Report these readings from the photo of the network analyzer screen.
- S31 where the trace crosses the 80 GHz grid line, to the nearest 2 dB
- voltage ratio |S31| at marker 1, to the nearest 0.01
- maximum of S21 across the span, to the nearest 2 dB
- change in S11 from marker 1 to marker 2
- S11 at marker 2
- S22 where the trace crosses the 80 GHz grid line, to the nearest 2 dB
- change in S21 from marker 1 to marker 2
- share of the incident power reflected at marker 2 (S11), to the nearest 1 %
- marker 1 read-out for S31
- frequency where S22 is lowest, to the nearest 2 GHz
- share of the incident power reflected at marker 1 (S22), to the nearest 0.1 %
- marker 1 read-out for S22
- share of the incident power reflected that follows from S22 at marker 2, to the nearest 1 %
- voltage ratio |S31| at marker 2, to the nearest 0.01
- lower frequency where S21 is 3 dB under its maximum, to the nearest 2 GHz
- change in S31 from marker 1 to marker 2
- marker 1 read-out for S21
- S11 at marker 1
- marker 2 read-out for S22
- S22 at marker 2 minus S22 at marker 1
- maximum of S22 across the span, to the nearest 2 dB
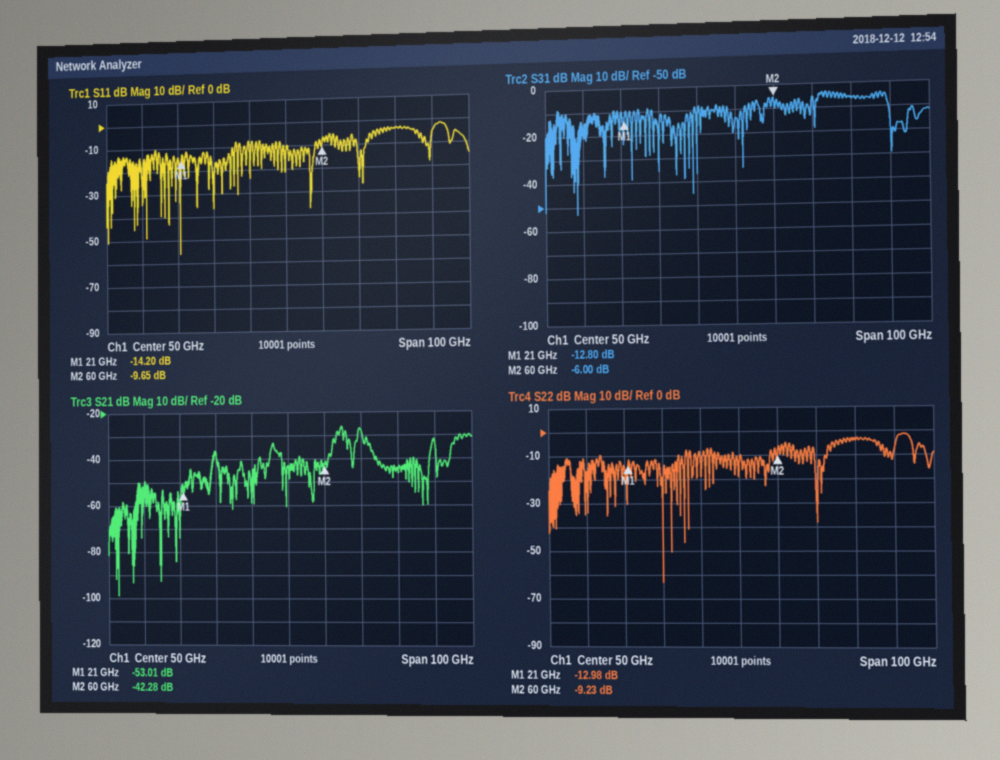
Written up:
-6 dB
0.23
-26 dB
4.55 dB
-9.65 dB
-4 dB
10.73 dB
11 %
-12.80 dB
30 GHz
5.0 %
-12.98 dB
12 %
0.50
64 GHz
6.80 dB
-53.01 dB
-14.20 dB
-9.23 dB
3.75 dB
-2 dB
